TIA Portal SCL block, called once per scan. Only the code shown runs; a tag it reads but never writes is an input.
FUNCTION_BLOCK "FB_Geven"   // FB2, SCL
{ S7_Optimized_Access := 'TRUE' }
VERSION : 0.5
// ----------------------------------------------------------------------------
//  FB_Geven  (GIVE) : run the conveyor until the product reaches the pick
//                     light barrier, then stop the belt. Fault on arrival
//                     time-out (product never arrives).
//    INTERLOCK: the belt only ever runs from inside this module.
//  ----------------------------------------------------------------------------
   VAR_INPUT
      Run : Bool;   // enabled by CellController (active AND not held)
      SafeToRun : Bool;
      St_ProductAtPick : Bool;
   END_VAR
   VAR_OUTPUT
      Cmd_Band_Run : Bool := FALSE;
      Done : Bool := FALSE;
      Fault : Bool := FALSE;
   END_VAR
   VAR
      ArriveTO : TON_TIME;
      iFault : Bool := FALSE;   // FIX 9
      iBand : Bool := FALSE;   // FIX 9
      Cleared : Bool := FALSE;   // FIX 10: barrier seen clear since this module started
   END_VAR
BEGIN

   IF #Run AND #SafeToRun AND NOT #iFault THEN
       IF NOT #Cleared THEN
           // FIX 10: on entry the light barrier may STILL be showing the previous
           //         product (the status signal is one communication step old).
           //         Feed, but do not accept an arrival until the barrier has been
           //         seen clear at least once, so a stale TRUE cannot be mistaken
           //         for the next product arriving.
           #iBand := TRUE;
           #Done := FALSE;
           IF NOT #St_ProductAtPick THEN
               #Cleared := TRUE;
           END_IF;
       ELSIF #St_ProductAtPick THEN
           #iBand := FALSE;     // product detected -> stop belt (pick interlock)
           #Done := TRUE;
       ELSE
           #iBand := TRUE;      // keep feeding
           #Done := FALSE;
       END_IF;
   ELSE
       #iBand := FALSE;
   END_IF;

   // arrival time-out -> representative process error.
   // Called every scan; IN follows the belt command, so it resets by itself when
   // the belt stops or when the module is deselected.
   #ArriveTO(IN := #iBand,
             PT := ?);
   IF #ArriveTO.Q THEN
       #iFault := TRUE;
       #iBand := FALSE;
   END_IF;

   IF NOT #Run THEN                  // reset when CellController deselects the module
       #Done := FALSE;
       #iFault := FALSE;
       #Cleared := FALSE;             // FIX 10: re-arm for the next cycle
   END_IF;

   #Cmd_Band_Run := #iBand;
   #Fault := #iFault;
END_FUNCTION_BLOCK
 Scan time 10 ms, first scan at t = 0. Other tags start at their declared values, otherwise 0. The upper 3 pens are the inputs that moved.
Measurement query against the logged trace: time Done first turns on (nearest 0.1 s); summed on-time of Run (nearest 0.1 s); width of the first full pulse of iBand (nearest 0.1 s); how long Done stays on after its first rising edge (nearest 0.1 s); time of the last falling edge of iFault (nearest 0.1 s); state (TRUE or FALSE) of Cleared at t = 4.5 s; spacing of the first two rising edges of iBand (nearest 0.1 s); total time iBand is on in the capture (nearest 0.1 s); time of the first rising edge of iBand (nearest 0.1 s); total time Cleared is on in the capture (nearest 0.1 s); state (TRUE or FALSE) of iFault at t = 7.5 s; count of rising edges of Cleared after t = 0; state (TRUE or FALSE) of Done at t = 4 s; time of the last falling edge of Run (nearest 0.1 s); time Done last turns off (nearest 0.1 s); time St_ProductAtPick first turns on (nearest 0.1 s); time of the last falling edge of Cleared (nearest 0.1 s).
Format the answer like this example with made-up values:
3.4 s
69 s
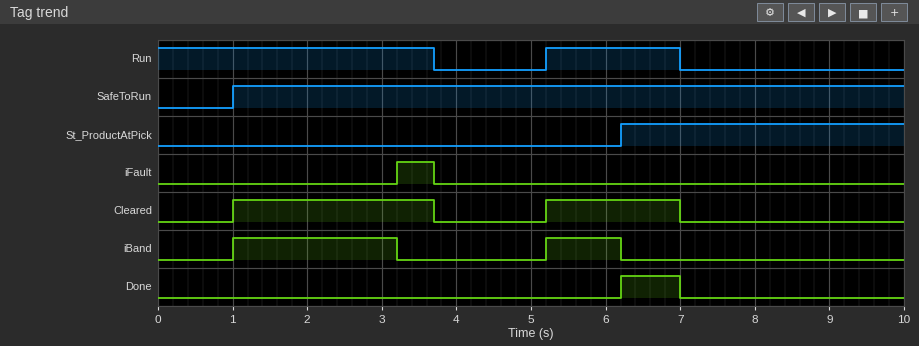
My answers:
6.2 s
5.5 s
2.2 s
0.8 s
3.7 s
FALSE
4.2 s
3.2 s
1.0 s
4.5 s
FALSE
2
FALSE
7.0 s
7.0 s
6.2 s
7.0 s
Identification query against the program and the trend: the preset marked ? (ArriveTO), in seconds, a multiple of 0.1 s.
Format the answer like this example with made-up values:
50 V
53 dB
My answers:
2.2 s
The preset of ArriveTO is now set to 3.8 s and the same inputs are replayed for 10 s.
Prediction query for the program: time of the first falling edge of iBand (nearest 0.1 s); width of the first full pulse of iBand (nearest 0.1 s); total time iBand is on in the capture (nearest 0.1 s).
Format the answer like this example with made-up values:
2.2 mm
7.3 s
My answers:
3.7 s
2.7 s
3.7 s
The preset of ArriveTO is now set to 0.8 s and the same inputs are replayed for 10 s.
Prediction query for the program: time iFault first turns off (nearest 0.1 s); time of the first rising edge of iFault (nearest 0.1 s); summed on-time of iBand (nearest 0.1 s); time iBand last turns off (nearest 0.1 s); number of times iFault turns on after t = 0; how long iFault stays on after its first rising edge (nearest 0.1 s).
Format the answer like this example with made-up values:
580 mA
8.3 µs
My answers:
3.7 s
1.8 s
1.6 s
6.0 s
2
1.9 s
